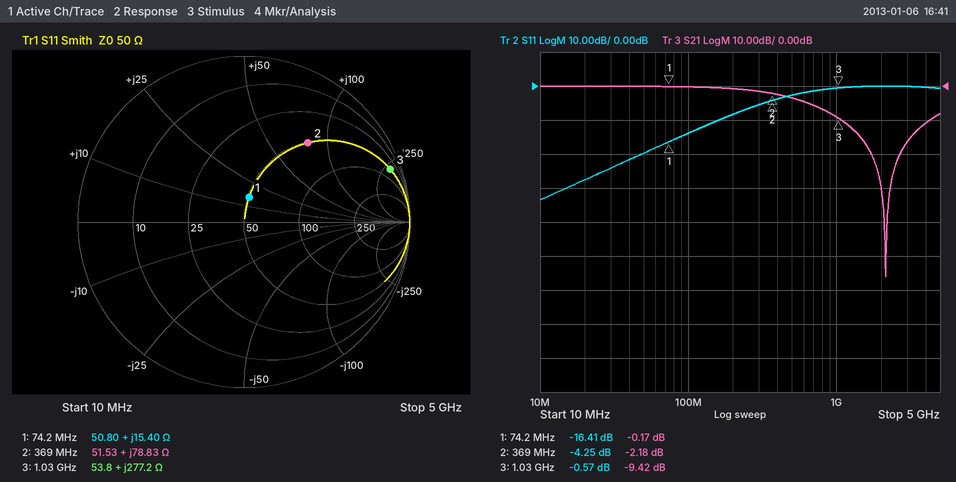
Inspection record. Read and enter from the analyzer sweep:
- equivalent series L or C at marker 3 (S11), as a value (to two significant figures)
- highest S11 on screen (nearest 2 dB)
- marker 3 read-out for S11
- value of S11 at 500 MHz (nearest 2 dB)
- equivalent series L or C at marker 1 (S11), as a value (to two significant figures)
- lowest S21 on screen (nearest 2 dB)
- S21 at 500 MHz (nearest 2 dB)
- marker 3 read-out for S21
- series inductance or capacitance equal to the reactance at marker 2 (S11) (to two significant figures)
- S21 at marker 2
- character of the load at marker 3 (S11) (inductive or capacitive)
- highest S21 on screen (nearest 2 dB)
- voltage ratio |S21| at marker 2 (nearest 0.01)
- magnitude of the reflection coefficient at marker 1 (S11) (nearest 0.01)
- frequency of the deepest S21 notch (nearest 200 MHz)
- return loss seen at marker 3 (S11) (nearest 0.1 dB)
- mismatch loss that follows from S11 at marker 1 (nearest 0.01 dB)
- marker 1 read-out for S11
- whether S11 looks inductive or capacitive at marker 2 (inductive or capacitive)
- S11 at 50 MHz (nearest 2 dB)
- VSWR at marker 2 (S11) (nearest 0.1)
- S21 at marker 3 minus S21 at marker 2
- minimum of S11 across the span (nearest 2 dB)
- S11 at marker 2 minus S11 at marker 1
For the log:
43 nH
0 dB
-0.57 dB
-2 dB
33 nH
-56 dB
-4 dB
-9.42 dB
34 nH
-2.18 dB
inductive
0 dB
0.78
0.15
2.2 GHz
0.6 dB
0.10 dB
-16.41 dB
inductive
-20 dB
4.2
-7.24 dB
-34 dB
12.16 dB
